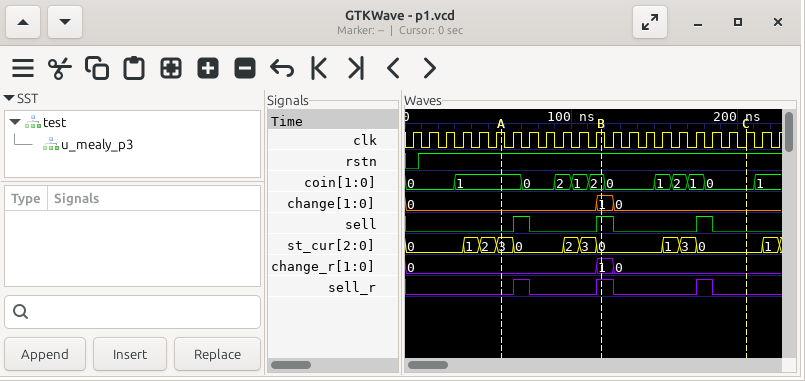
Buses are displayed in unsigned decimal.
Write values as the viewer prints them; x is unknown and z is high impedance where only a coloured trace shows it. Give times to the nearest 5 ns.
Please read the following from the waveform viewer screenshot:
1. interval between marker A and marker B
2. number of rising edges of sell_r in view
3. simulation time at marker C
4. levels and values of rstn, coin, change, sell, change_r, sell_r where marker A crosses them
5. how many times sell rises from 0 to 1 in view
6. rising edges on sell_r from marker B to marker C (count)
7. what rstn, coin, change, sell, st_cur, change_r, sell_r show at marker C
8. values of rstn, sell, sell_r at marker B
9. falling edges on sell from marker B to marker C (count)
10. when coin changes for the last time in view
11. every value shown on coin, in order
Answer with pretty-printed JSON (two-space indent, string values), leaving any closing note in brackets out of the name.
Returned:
{
  "interval between marker A and marker B": "60 ns",
  "number of rising edges of sell_r in view": "3",
  "simulation time at marker C": "205 ns",
  "levels and values of rstn, coin, change, sell, change_r, sell_r where marker A crosses them": "rstn=1, coin=1, change=0, sell=0, change_r=0, sell_r=0",
  "how many times sell rises from 0 to 1 in view": "3",
  "rising edges on sell_r from marker B to marker C": "1",
  "what rstn, coin, change, sell, st_cur, change_r, sell_r show at marker C": "rstn=1, coin=0, change=0, sell=0, st_cur=0, change_r=0, sell_r=0",
  "values of rstn, sell, sell_r at marker B": "rstn=1, sell=1, sell_r=1",
  "falling edges on sell from marker B to marker C": "2",
  "when coin changes for the last time in view": "210 ns",
  "every value shown on coin, in order": "0, 1, 0, 2, 1, 2, 0, 1, 2, 1, 0, 1"
}
